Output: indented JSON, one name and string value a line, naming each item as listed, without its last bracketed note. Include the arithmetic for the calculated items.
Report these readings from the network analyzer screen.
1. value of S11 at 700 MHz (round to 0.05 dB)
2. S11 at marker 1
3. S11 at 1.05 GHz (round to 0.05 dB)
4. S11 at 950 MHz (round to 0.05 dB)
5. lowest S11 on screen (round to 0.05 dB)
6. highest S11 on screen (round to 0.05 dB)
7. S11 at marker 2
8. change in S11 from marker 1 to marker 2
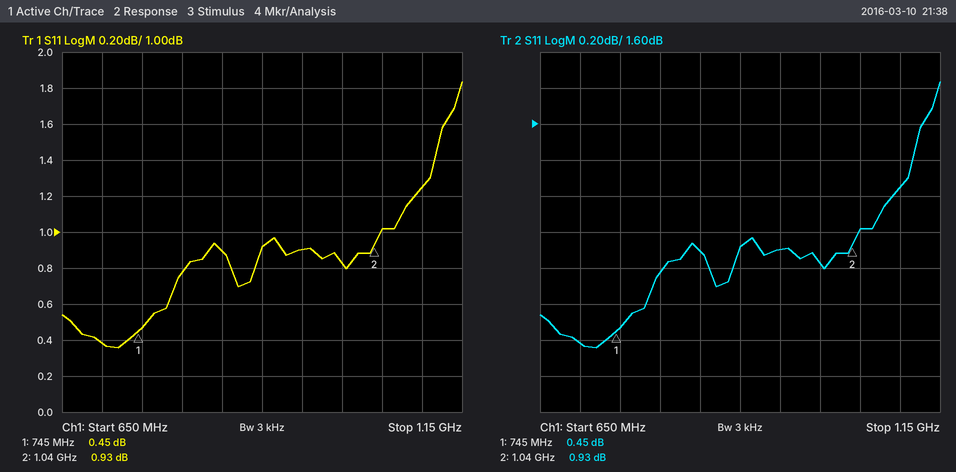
{
  "value of S11 at 700 MHz": "0.40 dB",
  "S11 at marker 1": "0.45 dB",
  "S11 at 1.05 GHz": "1.00 dB",
  "S11 at 950 MHz": "0.90 dB",
  "lowest S11 on screen": "0.35 dB",
  "highest S11 on screen": "1.85 dB",
  "S11 at marker 2": "0.93 dB",
  "change in S11 from marker 1 to marker 2": "0.93 − (0.45) = 0.48 dB"
}
